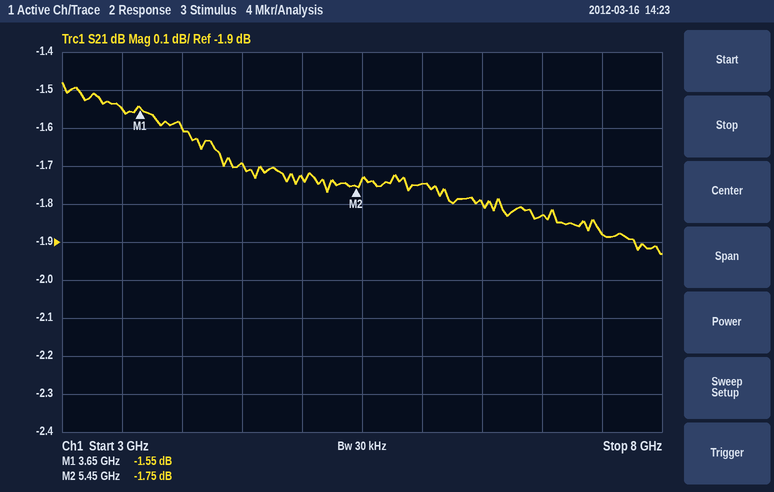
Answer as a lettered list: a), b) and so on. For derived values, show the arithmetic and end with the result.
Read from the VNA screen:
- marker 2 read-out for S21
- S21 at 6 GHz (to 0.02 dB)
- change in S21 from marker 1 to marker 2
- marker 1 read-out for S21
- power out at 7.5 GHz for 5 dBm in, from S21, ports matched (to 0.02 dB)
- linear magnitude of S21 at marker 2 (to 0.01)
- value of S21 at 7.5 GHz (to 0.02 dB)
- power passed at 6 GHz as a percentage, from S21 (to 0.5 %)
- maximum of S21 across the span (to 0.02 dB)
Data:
a) -1.75 dB
b) -1.74 dB
c) -1.75 − (-1.55) = -0.20 dB
d) -1.55 dB
e) 5 dBm + (-1.88 dB) = 3.12 dBm
f) 10^(-1.75/20) ≈ 0.82
g) -1.88 dB
h) 10^(-1.74/10) ≈ 67.0 %
i) -1.48 dB
